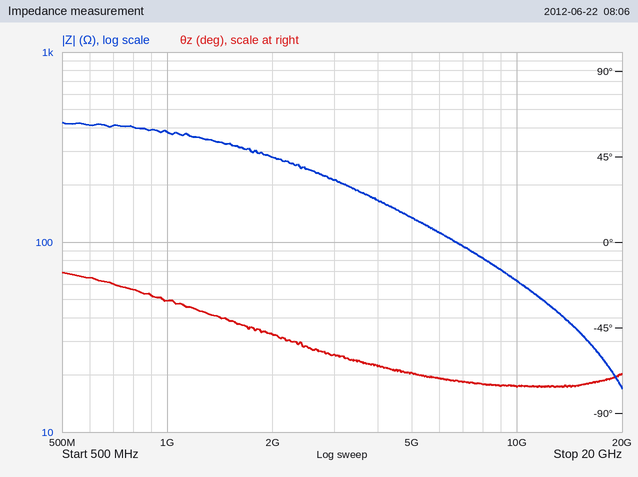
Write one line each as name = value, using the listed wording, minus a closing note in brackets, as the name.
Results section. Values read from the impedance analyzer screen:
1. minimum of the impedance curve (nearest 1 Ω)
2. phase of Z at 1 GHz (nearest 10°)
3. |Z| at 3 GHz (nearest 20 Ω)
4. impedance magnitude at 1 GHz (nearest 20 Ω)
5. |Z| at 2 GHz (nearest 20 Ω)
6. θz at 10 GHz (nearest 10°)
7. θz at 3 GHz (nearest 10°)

minimum of the impedance curve = 17 Ω
phase of Z at 1 GHz = -30°
|Z| at 3 GHz = 220 Ω
impedance magnitude at 1 GHz = 380 Ω
|Z| at 2 GHz = 280 Ω
θz at 10 GHz = -80°
θz at 3 GHz = -60°
